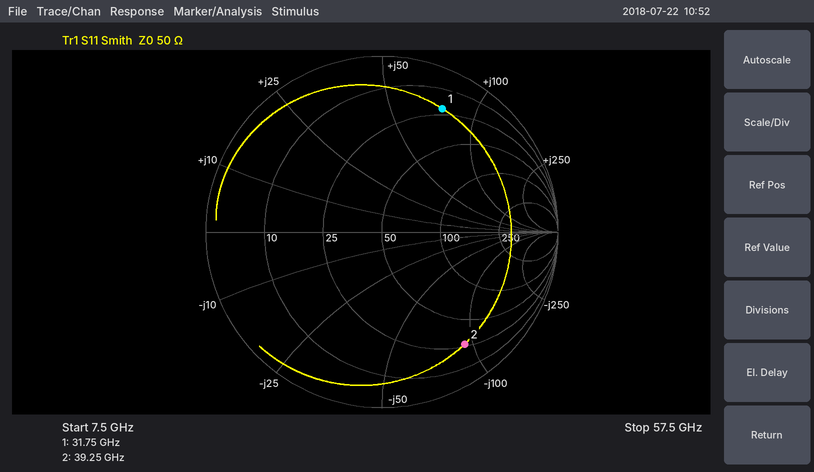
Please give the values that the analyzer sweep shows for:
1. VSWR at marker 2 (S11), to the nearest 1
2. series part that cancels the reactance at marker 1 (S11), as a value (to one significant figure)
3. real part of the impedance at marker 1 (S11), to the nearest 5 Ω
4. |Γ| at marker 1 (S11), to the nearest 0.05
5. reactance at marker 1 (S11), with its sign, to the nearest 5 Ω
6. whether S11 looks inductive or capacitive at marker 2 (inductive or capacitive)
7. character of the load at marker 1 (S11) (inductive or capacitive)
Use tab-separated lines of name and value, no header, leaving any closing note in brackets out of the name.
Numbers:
VSWR at marker 2 (S11), to the nearest 1	9
series part that cancels the reactance at marker 1 (S11), as a value	70 fF
real part of the impedance at marker 1 (S11), to the nearest 5 Ω	20 Ω
|Γ| at marker 1 (S11), to the nearest 0.05	0.80
reactance at marker 1 (S11), with its sign, to the nearest 5 Ω	+75 Ω
whether S11 looks inductive or capacitive at marker 2	capacitive
character of the load at marker 1 (S11)	inductive
